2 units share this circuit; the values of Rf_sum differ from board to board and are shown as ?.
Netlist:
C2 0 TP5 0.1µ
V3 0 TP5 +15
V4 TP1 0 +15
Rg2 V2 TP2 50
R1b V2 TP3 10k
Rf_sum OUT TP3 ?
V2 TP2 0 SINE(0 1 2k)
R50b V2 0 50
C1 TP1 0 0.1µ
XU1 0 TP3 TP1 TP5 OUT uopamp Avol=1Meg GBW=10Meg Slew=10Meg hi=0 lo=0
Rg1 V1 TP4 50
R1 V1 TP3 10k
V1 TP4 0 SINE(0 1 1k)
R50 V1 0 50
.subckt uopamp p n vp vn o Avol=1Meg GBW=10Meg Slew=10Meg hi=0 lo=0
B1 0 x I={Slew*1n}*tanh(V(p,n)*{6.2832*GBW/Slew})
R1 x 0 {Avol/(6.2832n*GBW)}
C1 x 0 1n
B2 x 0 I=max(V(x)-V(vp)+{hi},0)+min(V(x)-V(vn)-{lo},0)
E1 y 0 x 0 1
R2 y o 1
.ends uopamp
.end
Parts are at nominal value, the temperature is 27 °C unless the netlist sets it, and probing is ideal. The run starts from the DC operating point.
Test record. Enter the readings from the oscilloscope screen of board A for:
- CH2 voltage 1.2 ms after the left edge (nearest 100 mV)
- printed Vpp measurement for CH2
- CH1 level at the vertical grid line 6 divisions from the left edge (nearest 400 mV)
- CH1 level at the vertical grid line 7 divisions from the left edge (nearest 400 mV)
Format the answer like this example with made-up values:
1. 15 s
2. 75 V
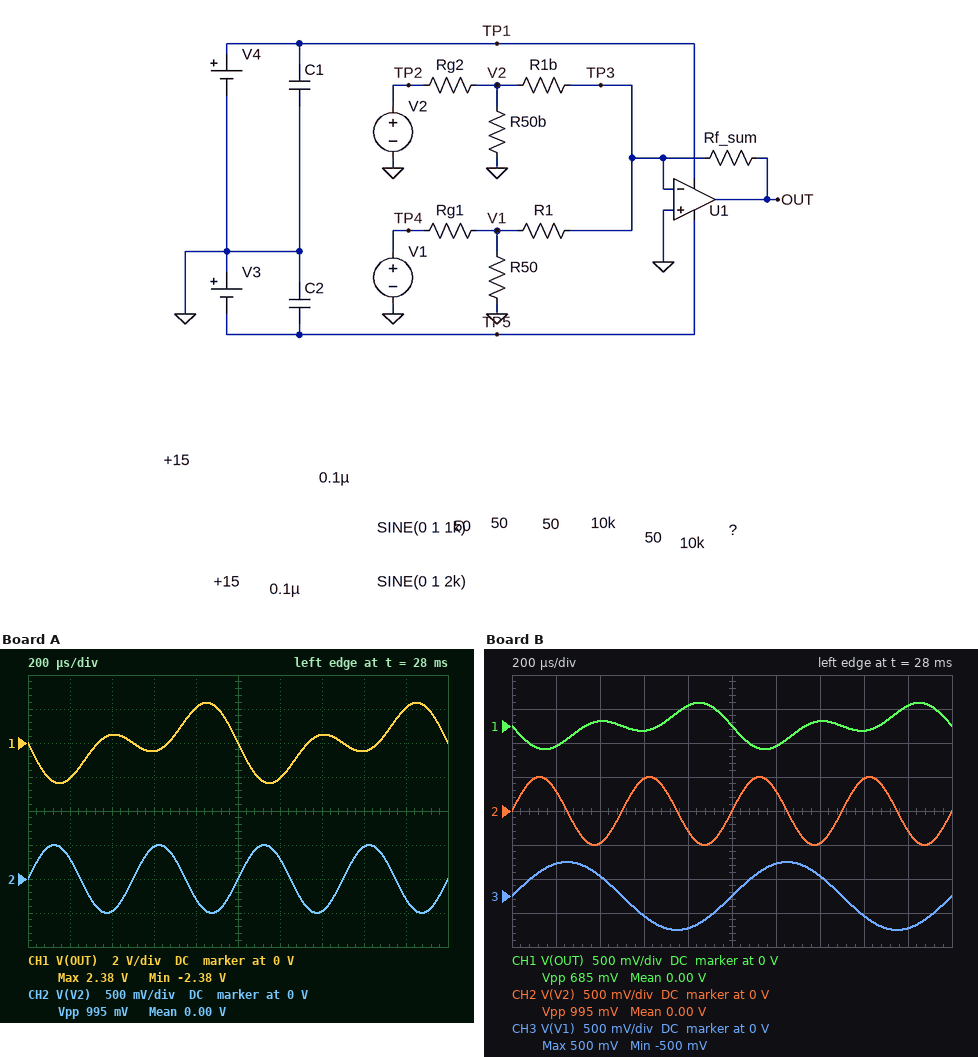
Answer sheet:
1. 300 mV
2. 995 mV
3. -2.0 V
4. 400 mV
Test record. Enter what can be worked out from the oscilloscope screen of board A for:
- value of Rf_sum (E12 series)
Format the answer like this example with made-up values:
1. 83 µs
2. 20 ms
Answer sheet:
1. 27 kΩ
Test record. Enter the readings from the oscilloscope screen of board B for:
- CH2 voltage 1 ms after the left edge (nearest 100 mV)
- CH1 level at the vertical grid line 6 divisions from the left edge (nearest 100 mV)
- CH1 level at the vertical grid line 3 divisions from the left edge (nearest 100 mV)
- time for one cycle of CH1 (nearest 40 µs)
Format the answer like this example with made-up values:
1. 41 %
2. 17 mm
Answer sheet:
1. 0 V
2. -300 mV
3. -100 mV
4. 1.00 ms
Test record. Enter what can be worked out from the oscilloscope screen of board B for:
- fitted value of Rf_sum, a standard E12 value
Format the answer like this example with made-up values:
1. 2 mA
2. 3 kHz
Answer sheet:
1. 3.9 kΩ
